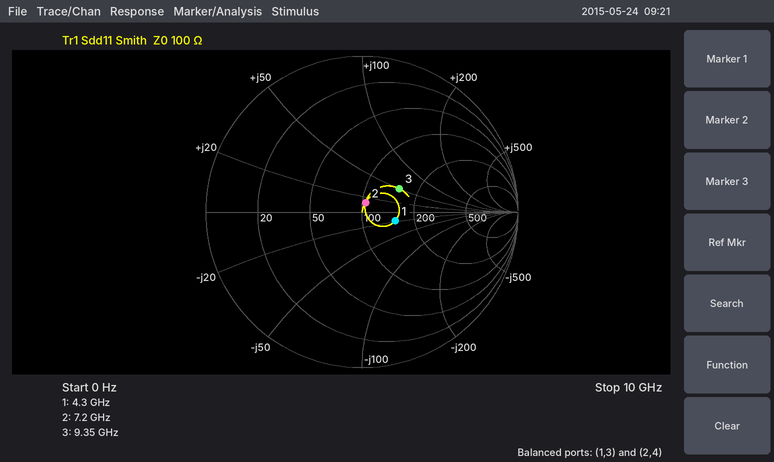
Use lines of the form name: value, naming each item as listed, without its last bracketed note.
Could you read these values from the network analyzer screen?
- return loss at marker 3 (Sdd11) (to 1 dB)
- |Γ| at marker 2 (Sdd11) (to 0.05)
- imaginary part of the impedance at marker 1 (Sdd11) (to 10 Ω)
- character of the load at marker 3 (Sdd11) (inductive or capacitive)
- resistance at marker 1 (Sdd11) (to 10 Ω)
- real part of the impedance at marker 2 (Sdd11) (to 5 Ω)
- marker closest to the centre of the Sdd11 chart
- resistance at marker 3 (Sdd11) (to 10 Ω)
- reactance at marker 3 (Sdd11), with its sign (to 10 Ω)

return loss at marker 3 (Sdd11): 11 dB
|Γ| at marker 2 (Sdd11): 0.05
imaginary part of the impedance at marker 1 (Sdd11): -20 Ω
character of the load at marker 3 (Sdd11): inductive
resistance at marker 1 (Sdd11): 150 Ω
real part of the impedance at marker 2 (Sdd11): 105 Ω
marker closest to the centre of the Sdd11 chart: marker 2
resistance at marker 3 (Sdd11): 150 Ω
reactance at marker 3 (Sdd11), with its sign: +50 Ω
